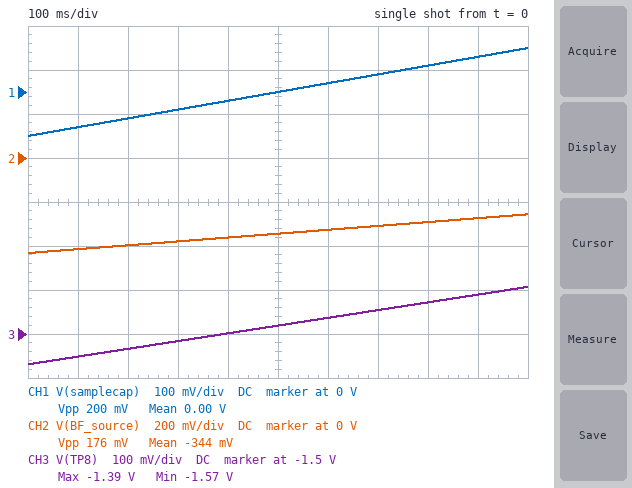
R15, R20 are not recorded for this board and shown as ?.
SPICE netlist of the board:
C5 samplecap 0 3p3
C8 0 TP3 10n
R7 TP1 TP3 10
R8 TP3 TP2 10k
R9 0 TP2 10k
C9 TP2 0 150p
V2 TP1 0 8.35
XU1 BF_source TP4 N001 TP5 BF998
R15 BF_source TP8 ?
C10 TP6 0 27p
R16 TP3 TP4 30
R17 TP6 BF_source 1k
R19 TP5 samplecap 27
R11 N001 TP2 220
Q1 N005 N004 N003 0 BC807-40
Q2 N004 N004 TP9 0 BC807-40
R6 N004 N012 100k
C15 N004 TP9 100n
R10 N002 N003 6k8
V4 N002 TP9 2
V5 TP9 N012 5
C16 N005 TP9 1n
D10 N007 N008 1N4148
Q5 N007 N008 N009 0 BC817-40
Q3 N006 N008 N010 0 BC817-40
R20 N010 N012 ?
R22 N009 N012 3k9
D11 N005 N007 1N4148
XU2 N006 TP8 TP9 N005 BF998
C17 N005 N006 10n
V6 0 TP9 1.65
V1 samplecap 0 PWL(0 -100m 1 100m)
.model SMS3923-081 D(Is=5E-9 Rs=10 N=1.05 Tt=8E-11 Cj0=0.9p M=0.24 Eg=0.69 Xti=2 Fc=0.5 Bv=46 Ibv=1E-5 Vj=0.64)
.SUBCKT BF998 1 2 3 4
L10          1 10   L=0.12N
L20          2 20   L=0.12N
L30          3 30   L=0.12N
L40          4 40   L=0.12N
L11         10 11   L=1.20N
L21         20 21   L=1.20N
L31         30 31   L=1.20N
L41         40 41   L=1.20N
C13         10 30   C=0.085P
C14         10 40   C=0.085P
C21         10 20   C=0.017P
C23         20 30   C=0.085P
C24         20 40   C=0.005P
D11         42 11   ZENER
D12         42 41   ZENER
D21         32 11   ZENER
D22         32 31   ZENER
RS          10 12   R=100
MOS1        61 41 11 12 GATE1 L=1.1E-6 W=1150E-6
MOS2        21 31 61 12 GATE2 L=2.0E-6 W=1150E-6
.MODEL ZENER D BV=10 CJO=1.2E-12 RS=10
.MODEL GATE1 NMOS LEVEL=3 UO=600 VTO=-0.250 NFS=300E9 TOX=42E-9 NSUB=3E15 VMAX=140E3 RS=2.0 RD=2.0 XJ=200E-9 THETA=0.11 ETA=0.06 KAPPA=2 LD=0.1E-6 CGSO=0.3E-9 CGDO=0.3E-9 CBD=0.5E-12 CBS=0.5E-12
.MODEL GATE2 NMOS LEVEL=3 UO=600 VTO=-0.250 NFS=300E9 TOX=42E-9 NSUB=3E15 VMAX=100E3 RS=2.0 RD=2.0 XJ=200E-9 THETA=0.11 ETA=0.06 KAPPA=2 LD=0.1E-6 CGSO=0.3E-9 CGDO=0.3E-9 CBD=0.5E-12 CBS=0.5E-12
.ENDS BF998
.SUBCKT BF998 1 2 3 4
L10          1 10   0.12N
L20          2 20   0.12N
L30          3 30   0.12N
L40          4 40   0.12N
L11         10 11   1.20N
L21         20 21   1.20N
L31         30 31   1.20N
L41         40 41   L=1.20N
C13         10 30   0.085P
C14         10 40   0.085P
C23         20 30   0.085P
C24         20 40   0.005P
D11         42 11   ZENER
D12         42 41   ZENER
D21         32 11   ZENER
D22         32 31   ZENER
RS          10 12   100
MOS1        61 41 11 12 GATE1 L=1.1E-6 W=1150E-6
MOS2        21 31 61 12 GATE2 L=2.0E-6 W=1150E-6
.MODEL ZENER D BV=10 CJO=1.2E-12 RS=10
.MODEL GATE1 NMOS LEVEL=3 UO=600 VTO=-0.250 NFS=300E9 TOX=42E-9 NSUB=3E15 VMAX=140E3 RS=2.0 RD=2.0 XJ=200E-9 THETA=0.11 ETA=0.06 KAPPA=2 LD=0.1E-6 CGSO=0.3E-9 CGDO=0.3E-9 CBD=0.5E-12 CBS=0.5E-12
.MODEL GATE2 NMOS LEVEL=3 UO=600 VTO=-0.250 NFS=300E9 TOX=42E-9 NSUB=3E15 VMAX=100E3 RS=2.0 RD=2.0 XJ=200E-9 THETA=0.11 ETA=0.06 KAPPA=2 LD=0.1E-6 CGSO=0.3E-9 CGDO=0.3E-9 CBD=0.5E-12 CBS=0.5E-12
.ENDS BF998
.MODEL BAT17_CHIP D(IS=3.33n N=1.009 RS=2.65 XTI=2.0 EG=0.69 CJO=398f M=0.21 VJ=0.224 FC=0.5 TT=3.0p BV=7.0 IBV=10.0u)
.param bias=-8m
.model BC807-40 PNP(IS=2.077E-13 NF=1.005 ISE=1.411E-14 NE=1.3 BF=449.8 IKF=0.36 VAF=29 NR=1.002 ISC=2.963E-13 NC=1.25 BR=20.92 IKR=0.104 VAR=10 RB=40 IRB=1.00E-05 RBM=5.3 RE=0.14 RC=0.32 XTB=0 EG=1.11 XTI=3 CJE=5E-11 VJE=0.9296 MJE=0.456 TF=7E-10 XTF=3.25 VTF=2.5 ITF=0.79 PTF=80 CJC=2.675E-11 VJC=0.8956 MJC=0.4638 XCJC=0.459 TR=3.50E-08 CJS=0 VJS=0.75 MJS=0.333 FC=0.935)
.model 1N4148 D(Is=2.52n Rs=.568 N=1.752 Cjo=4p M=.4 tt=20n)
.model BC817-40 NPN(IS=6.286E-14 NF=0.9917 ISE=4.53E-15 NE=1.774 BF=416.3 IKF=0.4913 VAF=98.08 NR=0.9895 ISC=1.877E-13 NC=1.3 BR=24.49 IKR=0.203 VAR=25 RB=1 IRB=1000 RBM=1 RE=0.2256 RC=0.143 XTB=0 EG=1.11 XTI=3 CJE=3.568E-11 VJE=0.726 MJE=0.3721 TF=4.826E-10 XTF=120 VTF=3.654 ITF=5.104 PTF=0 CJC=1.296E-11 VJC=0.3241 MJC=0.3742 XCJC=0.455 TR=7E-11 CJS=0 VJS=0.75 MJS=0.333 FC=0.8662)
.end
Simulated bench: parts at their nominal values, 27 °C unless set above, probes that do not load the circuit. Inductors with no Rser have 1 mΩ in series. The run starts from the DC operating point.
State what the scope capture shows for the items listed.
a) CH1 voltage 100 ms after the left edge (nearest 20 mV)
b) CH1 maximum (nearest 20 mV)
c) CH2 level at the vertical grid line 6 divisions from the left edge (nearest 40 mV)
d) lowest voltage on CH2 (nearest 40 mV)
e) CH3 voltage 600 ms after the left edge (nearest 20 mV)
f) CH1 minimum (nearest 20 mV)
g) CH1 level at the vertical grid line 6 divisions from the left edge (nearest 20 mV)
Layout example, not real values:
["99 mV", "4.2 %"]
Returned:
["-80 mV", "100 mV", "-320 mV", "-440 mV", "-1.46 V", "-100 mV", "20 mV"]
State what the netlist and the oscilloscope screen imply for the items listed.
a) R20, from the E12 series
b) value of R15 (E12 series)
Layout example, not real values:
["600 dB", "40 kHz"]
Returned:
["39 Ω", "56 Ω"]
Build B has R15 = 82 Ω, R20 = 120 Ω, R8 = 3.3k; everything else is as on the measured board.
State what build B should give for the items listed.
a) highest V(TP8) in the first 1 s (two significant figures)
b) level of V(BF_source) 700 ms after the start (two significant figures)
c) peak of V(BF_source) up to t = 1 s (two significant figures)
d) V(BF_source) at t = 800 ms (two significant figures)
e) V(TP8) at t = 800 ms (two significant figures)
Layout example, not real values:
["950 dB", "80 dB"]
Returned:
["-310 mV", "280 mV", "340 mV", "300 mV", "-350 mV"]
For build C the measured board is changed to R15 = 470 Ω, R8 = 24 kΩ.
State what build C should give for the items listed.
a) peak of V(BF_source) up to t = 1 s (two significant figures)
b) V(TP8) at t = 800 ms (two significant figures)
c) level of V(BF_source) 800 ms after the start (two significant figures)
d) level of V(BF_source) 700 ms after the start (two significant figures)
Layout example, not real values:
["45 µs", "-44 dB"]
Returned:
["-160 mV", "-5.8 V", "-190 mV", "-210 mV"]
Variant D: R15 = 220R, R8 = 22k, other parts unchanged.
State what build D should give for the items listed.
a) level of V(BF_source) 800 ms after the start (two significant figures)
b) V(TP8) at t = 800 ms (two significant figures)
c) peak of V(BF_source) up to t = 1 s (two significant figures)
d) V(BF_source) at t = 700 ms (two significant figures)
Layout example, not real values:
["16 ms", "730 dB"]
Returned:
["-460 mV", "-4.9 V", "-430 mV", "-480 mV"]
